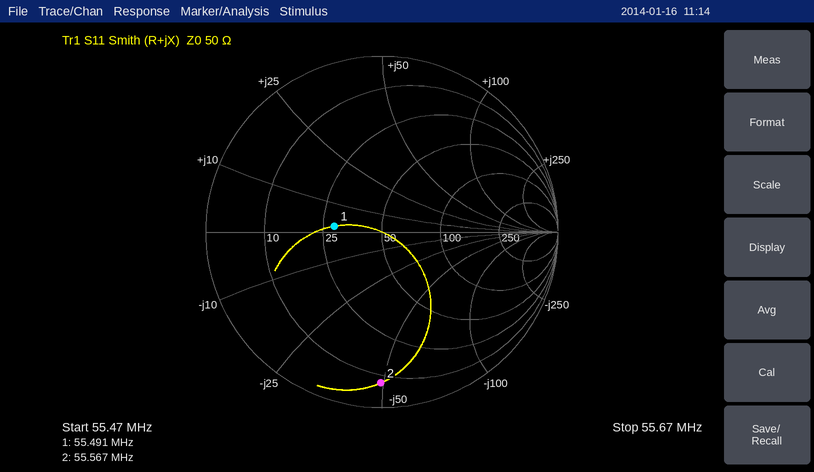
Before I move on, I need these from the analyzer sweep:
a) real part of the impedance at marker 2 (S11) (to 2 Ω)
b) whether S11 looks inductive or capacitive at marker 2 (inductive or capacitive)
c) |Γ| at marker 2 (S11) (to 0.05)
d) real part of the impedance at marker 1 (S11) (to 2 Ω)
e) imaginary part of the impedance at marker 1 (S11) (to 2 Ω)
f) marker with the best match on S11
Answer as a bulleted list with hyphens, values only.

- 8 Ω
- capacitive
- 0.85
- 28 Ω
- +2 Ω
- marker 1
